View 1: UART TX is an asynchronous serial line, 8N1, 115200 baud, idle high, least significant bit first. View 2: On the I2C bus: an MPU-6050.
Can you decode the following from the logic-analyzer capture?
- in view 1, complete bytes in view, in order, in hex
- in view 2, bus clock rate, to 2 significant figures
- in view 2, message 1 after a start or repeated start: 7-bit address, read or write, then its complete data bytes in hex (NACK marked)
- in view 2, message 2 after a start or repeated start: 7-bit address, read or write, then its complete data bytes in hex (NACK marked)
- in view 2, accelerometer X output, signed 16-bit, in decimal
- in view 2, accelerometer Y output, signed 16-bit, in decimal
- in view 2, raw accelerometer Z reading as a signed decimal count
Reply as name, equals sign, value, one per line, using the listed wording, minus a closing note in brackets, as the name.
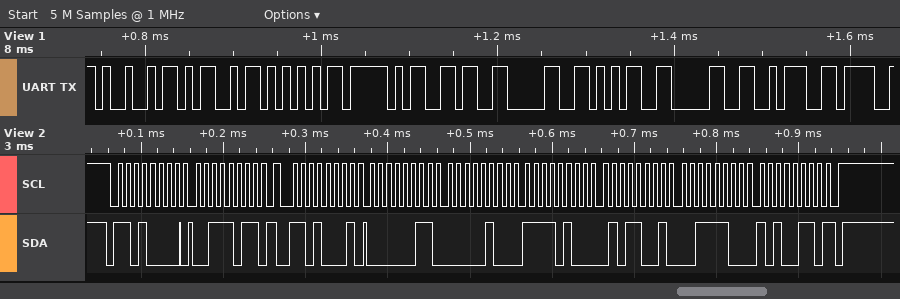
in view 1, complete bytes in view, in order, in hex = 0x49 0x4D 0x55 0x5F 0x36 0x30 0x35 0x30 0x3A
in view 2, bus clock rate, to 2 significant figures = 100 kHz
in view 2, message 1 after a start or repeated start: 7-bit address, read or write, then its complete data bytes in hex = 0x68 write: 3B
in view 2, message 2 after a start or repeated start: 7-bit address, read or write, then its complete data bytes in hex = 0x68 read: 03 04 F4 59 3C A6 NACK
in view 2, accelerometer X output, signed 16-bit, in decimal = 772
in view 2, accelerometer Y output, signed 16-bit, in decimal = -2983
in view 2, raw accelerometer Z reading as a signed decimal count = 15526
